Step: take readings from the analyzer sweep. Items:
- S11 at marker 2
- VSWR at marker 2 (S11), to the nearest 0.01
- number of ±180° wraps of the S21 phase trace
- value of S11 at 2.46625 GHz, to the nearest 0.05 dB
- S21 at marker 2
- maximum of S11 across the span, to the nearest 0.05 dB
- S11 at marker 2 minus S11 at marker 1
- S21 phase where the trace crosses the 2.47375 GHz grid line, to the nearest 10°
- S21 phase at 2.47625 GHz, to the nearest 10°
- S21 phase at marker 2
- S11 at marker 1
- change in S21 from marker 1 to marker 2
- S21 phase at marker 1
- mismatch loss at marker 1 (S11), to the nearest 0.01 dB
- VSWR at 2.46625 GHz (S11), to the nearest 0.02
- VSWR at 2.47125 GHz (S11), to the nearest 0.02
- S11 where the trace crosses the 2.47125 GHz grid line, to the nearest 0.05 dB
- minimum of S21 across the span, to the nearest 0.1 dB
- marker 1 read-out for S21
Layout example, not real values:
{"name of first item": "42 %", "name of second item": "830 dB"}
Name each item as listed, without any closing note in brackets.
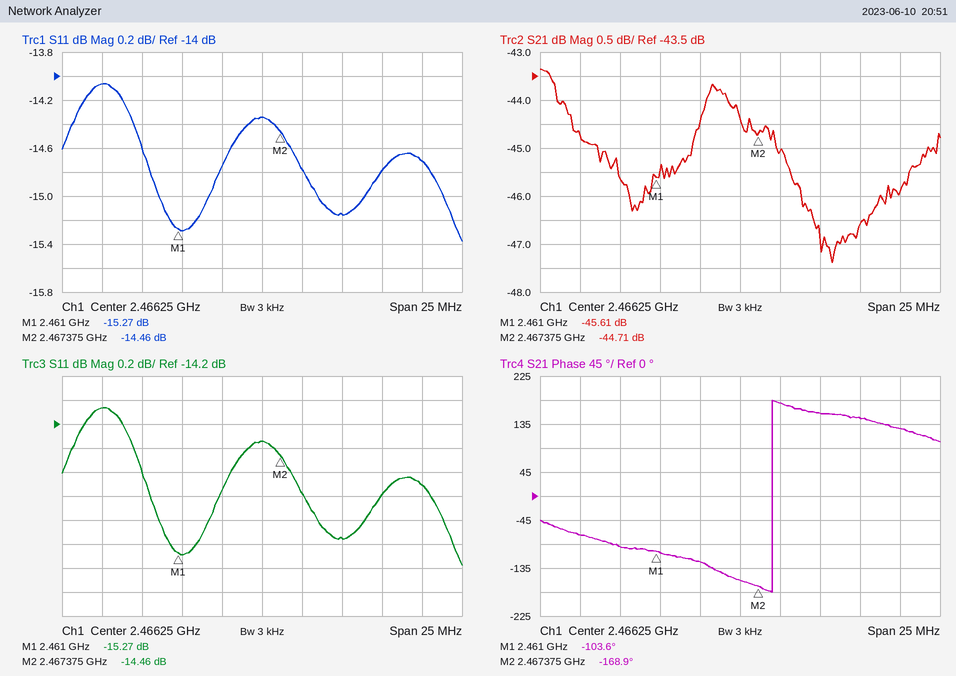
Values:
{"S11 at marker 2": "-14.46 dB", "VSWR at marker 2 (S11), to the nearest 0.01": "1.47", "number of ±180° wraps of the S21 phase trace": "1", "value of S11 at 2.46625 GHz, to the nearest 0.05 dB": "-14.35 dB", "S21 at marker 2": "-44.71 dB", "maximum of S11 across the span, to the nearest 0.05 dB": "-14.05 dB", "S11 at marker 2 minus S11 at marker 1": "0.81 dB", "S21 phase where the trace crosses the 2.47375 GHz grid line, to the nearest 10°": "150°", "S21 phase at 2.47625 GHz, to the nearest 10°": "130°", "S21 phase at marker 2": "-168.9°", "S11 at marker 1": "-15.27 dB", "change in S21 from marker 1 to marker 2": "0.90 dB", "S21 phase at marker 1": "-103.6°", "mismatch loss at marker 1 (S11), to the nearest 0.01 dB": "0.13 dB", "VSWR at 2.46625 GHz (S11), to the nearest 0.02": "1.48", "VSWR at 2.47125 GHz (S11), to the nearest 0.02": "1.42", "S11 where the trace crosses the 2.47125 GHz grid line, to the nearest 0.05 dB": "-15.15 dB", "minimum of S21 across the span, to the nearest 0.1 dB": "-47.4 dB", "marker 1 read-out for S21": "-45.61 dB"}
